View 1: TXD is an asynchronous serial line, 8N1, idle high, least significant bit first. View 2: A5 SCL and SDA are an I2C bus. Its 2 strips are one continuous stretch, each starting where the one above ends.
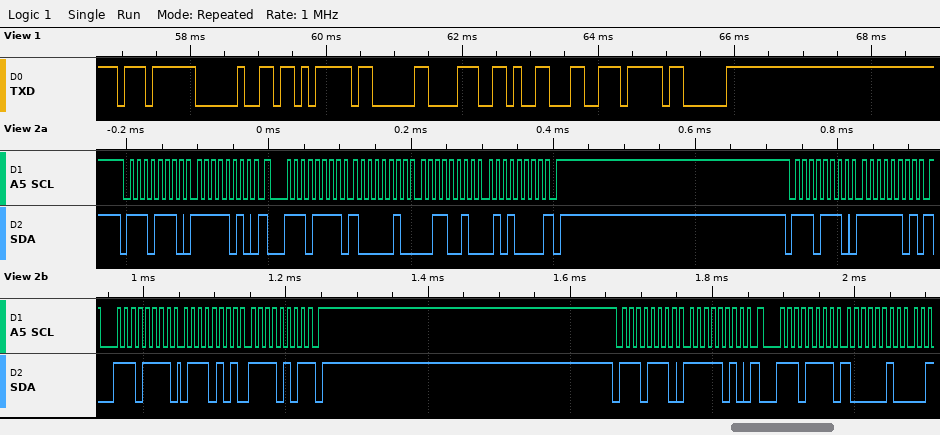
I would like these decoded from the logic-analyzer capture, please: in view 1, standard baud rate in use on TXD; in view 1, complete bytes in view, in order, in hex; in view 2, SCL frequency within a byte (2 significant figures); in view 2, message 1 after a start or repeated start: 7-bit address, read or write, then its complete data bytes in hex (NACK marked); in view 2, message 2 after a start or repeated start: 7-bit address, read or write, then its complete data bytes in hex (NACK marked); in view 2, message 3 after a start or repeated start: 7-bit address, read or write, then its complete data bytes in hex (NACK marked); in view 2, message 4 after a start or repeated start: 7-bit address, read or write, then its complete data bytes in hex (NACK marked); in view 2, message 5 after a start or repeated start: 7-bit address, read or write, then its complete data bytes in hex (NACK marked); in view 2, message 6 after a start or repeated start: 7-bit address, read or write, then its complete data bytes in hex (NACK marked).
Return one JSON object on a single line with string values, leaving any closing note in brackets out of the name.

{"in view 1, standard baud rate in use on TXD": "9600 baud", "in view 1, complete bytes in view, in order, in hex": "F7 20 EB 03 38 19 EE 03", "in view 2, SCL frequency within a byte": "100 kHz", "in view 2, message 1 after a start or repeated start: 7-bit address, read or write, then its complete data bytes in hex": "0x77 write: FA", "in view 2, message 2 after a start or repeated start: 7-bit address, read or write, then its complete data bytes in hex": "0x77 read: 82 32 50 NACK", "in view 2, message 3 after a start or repeated start: 7-bit address, read or write, then its complete data bytes in hex": "0x77 write: FD", "in view 2, message 4 after a start or repeated start: 7-bit address, read or write, then its complete data bytes in hex": "0x77 read: 75 F5 NACK", "in view 2, message 5 after a start or repeated start: 7-bit address, read or write, then its complete data bytes in hex": "0x77 write: FA", "in view 2, message 6 after a start or repeated start: 7-bit address, read or write, then its complete data bytes in hex": "0x77 read: 82"}
